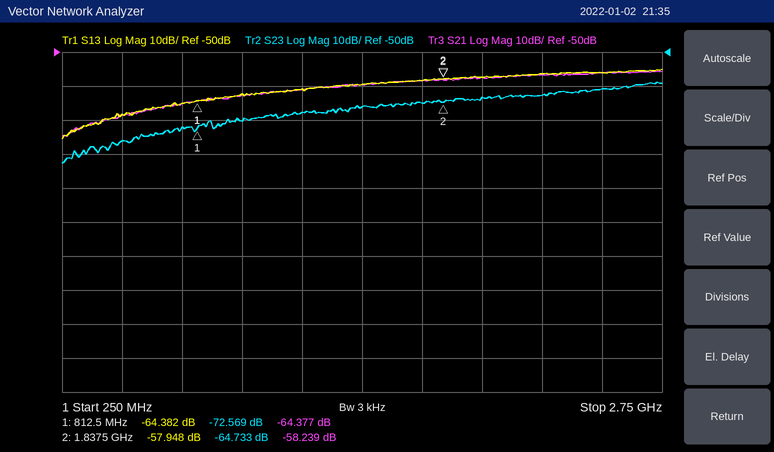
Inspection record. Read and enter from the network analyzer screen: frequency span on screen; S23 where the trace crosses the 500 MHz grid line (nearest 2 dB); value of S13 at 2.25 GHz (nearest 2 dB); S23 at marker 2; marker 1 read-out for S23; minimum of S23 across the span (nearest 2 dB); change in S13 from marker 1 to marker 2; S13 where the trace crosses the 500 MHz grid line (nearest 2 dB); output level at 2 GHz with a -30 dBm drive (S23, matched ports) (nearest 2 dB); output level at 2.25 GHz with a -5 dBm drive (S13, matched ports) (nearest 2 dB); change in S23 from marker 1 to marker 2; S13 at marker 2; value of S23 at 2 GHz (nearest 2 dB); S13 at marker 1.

2.5 GHz
-76 dB
-56 dB
-64.733 dB
-72.569 dB
-82 dB
6.434 dB
-68 dB
-94 dBm
-62 dBm
7.836 dB
-57.948 dB
-64 dB
-64.382 dB
